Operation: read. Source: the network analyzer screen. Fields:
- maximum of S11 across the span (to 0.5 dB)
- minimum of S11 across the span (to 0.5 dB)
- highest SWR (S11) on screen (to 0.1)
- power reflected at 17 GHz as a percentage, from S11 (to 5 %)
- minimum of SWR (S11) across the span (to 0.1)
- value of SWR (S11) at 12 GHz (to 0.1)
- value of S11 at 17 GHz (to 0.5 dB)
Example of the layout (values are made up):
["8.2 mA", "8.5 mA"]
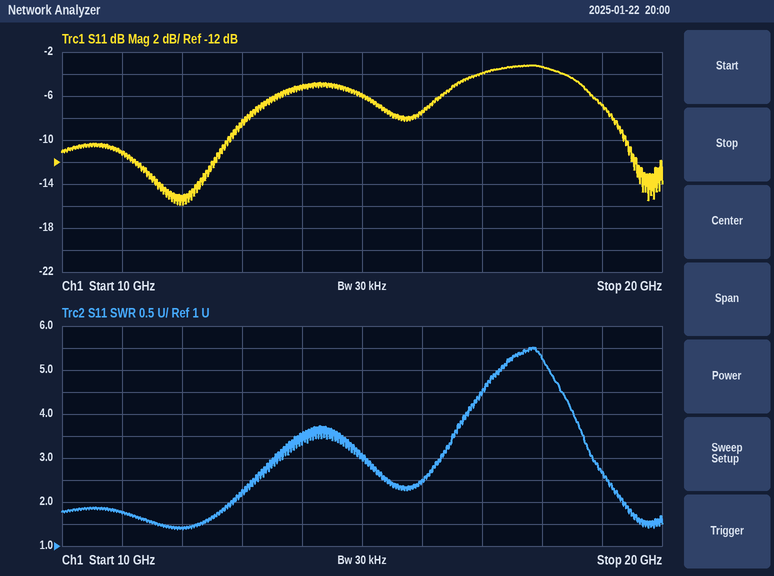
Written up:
["-3.0 dB", "-16.0 dB", "5.5", "40 %", "1.4", "1.4", "-4.0 dB"]
